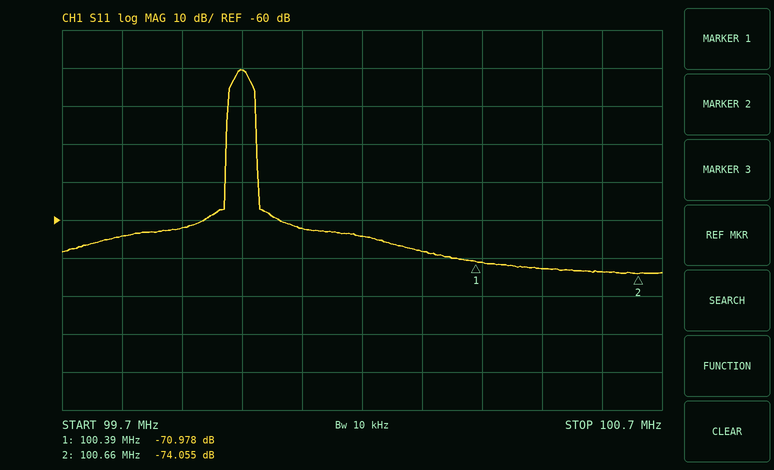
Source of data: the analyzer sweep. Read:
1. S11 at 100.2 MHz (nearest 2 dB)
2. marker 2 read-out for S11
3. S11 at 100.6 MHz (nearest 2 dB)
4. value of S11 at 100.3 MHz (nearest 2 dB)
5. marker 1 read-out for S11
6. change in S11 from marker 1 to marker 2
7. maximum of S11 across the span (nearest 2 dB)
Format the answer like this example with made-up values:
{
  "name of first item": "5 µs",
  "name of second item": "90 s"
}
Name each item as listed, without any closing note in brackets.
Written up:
{
  "S11 at 100.2 MHz": "-64 dB",
  "marker 2 read-out for S11": "-74.055 dB",
  "S11 at 100.6 MHz": "-74 dB",
  "value of S11 at 100.3 MHz": "-68 dB",
  "marker 1 read-out for S11": "-70.978 dB",
  "change in S11 from marker 1 to marker 2": "-3.077 dB",
  "maximum of S11 across the span": "-20 dB"
}
